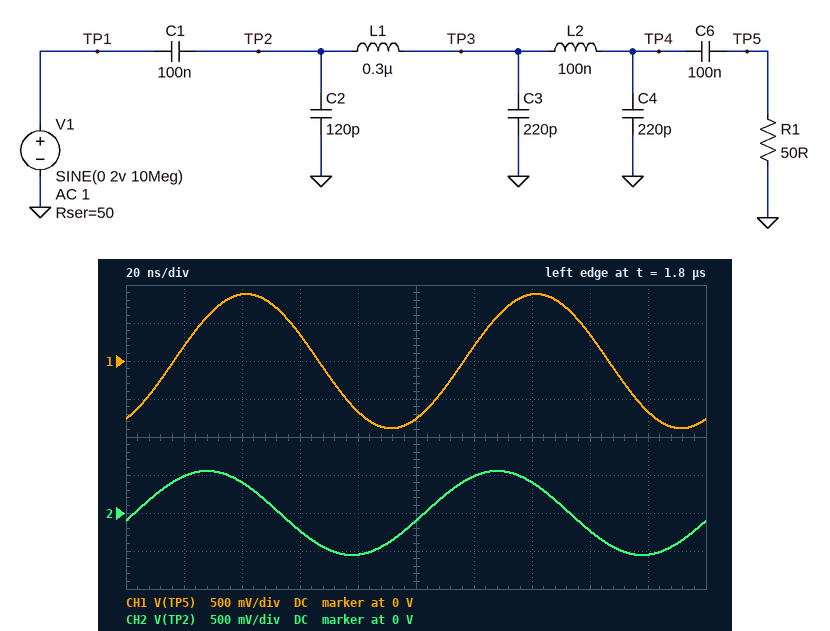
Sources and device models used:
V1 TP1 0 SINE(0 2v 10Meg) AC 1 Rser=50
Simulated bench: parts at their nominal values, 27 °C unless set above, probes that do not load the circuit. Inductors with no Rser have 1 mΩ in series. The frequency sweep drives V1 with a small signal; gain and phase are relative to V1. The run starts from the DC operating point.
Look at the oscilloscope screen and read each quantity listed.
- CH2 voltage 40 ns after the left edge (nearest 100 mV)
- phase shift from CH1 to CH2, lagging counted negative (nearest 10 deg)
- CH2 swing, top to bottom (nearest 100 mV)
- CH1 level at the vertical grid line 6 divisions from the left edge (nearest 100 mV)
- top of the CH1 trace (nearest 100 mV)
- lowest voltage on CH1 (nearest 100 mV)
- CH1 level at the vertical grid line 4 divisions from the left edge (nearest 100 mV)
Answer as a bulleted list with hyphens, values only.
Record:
- 400 mV
- 50 deg
- 1.1 V
- 200 mV
- 900 mV
- -900 mV
- -700 mV
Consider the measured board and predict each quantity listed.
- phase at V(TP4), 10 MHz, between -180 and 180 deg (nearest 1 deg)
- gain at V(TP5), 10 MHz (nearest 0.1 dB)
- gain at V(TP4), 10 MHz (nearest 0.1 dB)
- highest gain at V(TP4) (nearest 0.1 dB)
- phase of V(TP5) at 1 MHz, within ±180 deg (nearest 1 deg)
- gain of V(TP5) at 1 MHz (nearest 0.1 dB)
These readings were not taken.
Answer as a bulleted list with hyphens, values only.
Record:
- -59 deg
- -7.1 dB
- -7.1 dB
- -6.0 dB
- -5 deg
- -6.1 dB
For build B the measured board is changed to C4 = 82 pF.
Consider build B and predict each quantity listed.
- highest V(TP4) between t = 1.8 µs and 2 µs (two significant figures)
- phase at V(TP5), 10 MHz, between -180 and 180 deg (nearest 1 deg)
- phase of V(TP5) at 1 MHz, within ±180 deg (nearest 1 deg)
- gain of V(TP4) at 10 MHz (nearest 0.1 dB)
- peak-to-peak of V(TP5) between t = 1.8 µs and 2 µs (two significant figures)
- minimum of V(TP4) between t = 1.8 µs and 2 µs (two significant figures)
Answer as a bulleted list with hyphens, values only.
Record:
- 940 mV
- -50 deg
- -3 deg
- -6.5 dB
- 1.9 V
- -940 mV
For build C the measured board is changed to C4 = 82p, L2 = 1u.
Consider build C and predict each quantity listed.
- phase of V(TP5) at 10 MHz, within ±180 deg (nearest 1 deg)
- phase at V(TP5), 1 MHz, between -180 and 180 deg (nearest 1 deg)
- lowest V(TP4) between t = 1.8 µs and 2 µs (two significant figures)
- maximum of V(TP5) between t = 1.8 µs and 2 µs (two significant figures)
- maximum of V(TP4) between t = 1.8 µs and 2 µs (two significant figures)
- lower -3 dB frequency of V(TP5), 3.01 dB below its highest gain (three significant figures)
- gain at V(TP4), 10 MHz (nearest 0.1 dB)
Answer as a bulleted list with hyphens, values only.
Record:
- -89 deg
- -7 deg
- -920 mV
- 910 mV
- 920 mV
- 31.9 kHz
- -6.8 dB
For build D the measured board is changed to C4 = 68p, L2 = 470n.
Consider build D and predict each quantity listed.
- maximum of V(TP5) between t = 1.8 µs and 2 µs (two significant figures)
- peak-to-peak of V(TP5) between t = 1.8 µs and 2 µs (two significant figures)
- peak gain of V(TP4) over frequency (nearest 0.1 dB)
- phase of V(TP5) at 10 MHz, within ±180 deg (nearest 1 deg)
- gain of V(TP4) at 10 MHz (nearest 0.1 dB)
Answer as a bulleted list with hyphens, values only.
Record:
- 980 mV
- 2.0 V
- -6.0 dB
- -65 deg
- -6.2 dB
